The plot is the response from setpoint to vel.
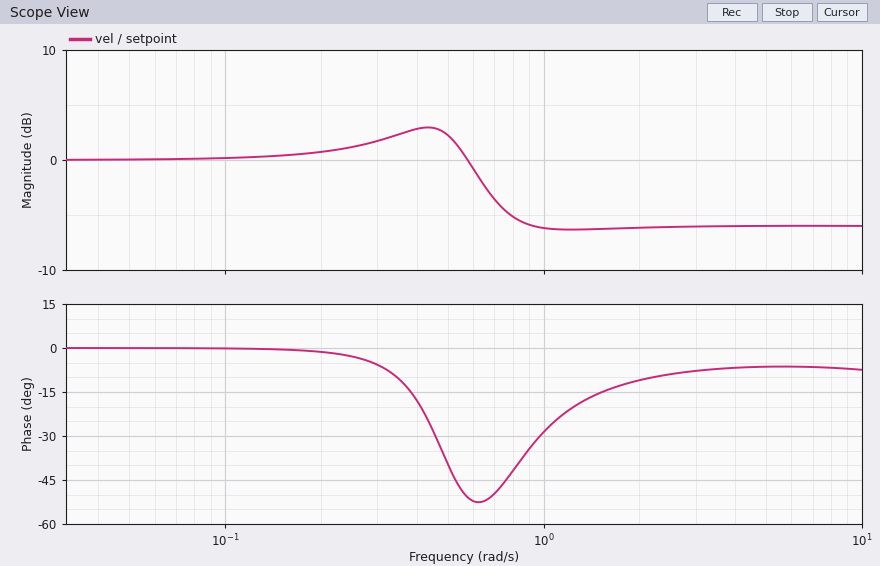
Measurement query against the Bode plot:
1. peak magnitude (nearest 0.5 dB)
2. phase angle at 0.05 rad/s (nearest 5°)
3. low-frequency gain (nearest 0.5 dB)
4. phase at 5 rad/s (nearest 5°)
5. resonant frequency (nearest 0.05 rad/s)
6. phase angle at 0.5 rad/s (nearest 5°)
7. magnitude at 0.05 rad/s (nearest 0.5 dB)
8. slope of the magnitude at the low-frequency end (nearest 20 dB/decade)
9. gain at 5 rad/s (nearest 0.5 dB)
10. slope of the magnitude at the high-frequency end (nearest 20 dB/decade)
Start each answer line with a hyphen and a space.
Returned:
- 3.0 dB
- 0°
- 0.0 dB
- -5°
- 0.45 rad/s
- -40°
- 0.0 dB
- 0 dB/decade
- -6.0 dB
- 0 dB/decade
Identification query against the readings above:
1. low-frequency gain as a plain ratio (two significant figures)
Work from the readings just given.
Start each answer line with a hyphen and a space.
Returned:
- 1.0
